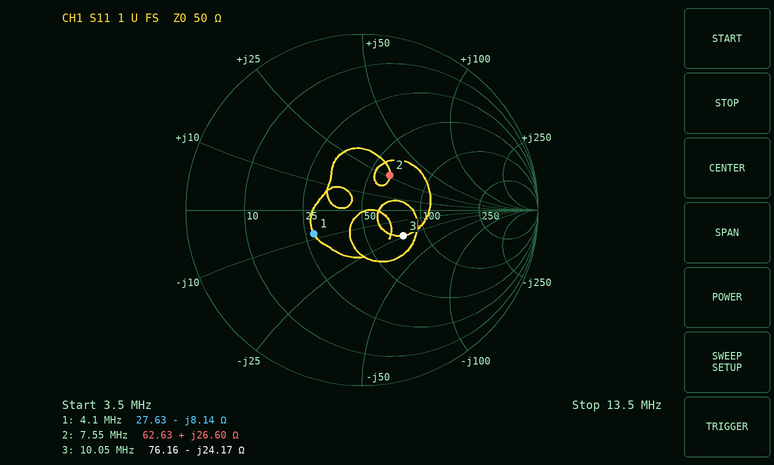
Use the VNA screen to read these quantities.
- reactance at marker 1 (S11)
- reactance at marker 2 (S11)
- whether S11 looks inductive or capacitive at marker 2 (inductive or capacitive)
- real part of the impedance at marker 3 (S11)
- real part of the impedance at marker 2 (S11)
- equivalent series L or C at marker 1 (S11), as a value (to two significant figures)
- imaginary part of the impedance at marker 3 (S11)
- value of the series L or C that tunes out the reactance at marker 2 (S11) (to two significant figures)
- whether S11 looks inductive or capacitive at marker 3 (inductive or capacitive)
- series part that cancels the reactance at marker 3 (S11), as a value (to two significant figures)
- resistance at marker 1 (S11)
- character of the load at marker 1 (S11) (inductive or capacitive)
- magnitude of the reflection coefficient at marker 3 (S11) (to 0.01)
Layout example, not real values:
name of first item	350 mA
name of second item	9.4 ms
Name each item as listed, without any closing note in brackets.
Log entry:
reactance at marker 1	-8.14 Ω
reactance at marker 2	+26.60 Ω
whether S11 looks inductive or capacitive at marker 2	inductive
real part of the impedance at marker 3	76.16 Ω
real part of the impedance at marker 2	62.63 Ω
equivalent series L or C at marker 1 (S11), as a value	4.8 nF
imaginary part of the impedance at marker 3	-24.17 Ω
value of the series L or C that tunes out the reactance at marker 2 (S11)	790 pF
whether S11 looks inductive or capacitive at marker 3	capacitive
series part that cancels the reactance at marker 3 (S11), as a value	380 nH
resistance at marker 1	27.63 Ω
character of the load at marker 1 (S11)	capacitive
magnitude of the reflection coefficient at marker 3 (S11)	0.28
